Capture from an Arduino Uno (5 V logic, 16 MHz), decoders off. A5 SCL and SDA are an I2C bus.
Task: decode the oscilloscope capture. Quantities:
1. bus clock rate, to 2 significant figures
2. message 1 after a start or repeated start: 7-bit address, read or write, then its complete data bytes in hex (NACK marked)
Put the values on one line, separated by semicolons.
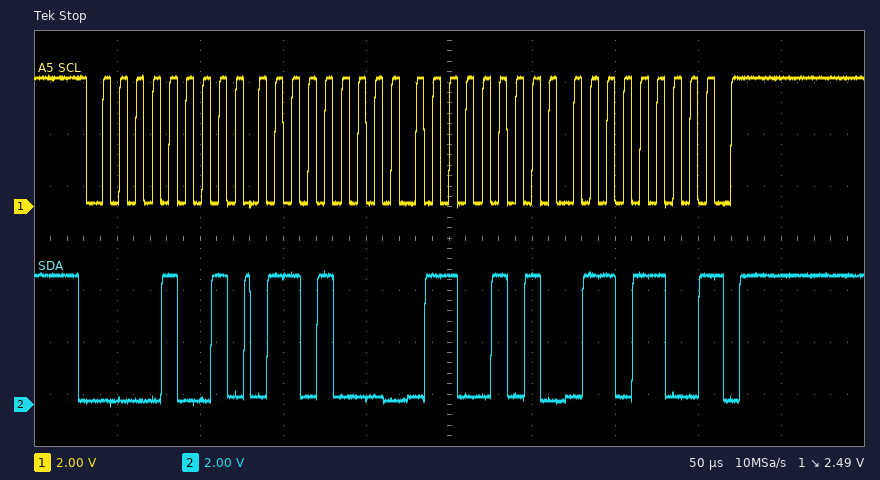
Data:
100 kHz; 0x04 read: 68 65 6C NACK
